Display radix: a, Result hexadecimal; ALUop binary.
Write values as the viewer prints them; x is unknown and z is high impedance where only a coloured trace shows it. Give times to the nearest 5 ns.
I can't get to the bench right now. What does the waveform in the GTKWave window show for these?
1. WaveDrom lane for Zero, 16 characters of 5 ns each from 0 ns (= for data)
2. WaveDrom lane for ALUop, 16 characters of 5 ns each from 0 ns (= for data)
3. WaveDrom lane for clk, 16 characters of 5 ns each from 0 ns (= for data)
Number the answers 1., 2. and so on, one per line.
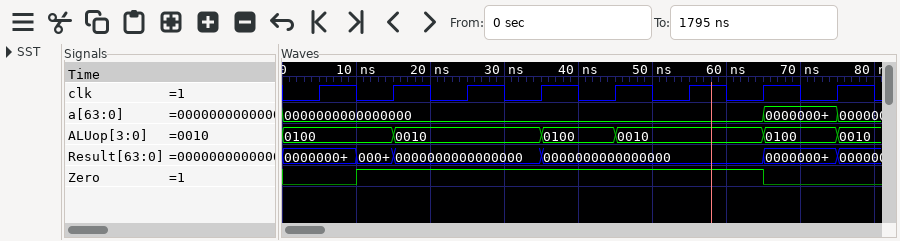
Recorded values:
1. {name: 'Zero', wave: '0.1..........0..'}
2. {name: 'ALUop', wave: '=..=...=.=...=.=', data: '0100 0010 0100 0010 0100 0010'}
3. {name: 'clk', wave: '0101010101010101'}
